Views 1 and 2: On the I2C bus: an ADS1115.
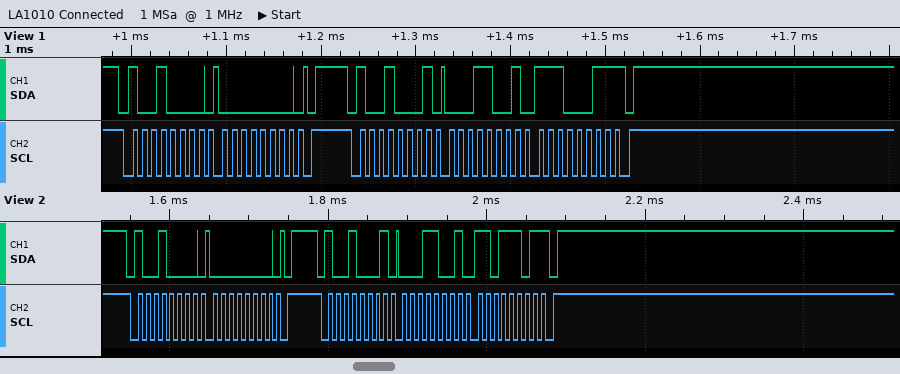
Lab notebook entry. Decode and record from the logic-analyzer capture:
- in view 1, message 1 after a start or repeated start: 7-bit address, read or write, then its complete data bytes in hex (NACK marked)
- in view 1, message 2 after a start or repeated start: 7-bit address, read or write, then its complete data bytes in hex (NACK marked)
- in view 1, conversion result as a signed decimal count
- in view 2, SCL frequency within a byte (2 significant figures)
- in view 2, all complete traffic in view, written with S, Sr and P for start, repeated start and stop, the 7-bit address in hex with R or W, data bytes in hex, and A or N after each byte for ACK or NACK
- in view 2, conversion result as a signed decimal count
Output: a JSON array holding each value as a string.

["0x48 write: 00", "0x48 read: 19 E3 NACK", "6627", "100 kHz", "S 48W A 00 A P S 48R A 19 A DD N P", "6621"]
